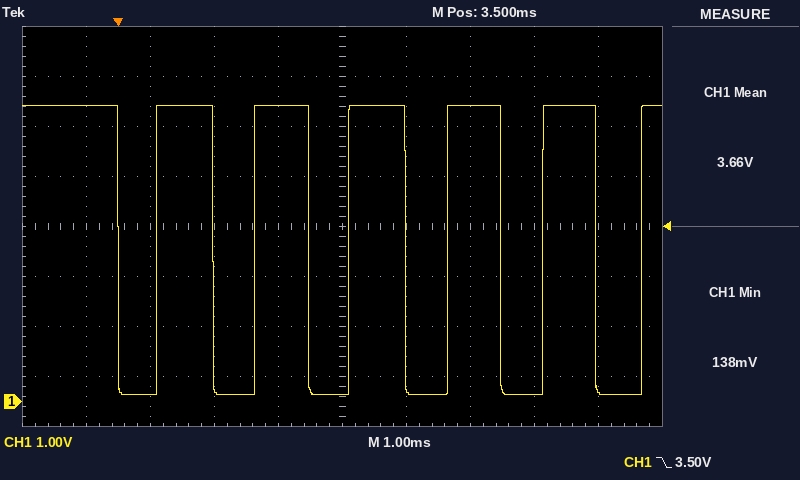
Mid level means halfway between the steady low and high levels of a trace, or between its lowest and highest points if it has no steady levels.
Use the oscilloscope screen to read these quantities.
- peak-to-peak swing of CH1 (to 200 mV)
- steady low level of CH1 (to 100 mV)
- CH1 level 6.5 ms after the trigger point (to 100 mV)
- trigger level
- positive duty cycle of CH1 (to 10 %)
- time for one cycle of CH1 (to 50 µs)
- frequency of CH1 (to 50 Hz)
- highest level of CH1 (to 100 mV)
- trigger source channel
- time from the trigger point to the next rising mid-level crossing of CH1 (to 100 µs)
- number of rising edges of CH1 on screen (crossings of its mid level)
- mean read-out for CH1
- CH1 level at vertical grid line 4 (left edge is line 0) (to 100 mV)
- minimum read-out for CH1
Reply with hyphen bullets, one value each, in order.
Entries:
- 5.8 V
- 100 mV
- 100 mV
- 3.50 V
- 60 %
- 1.50 ms
- 650 Hz
- 5.9 V
- CH1
- 600 µs
- 6
- 3.66 V
- 5.9 V
- 138 mV
